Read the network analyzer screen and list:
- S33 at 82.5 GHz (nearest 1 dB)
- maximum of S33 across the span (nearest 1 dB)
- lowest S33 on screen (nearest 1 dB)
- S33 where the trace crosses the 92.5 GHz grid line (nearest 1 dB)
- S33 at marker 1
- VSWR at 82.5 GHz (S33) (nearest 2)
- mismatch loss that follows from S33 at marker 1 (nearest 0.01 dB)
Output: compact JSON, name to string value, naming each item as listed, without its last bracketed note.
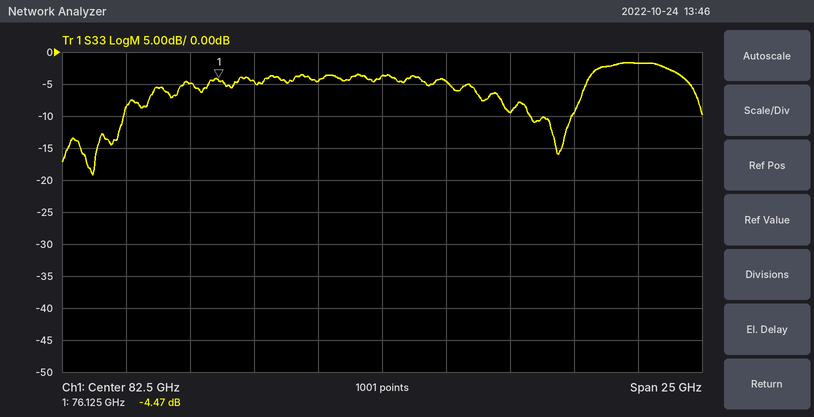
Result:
{"S33 at 82.5 GHz": "-4 dB", "maximum of S33 across the span": "-2 dB", "lowest S33 on screen": "-19 dB", "S33 where the trace crosses the 92.5 GHz grid line": "-2 dB", "S33 at marker 1": "-4.47 dB", "VSWR at 82.5 GHz (S33)": "4", "mismatch loss that follows from S33 at marker 1": "1.92 dB"}
